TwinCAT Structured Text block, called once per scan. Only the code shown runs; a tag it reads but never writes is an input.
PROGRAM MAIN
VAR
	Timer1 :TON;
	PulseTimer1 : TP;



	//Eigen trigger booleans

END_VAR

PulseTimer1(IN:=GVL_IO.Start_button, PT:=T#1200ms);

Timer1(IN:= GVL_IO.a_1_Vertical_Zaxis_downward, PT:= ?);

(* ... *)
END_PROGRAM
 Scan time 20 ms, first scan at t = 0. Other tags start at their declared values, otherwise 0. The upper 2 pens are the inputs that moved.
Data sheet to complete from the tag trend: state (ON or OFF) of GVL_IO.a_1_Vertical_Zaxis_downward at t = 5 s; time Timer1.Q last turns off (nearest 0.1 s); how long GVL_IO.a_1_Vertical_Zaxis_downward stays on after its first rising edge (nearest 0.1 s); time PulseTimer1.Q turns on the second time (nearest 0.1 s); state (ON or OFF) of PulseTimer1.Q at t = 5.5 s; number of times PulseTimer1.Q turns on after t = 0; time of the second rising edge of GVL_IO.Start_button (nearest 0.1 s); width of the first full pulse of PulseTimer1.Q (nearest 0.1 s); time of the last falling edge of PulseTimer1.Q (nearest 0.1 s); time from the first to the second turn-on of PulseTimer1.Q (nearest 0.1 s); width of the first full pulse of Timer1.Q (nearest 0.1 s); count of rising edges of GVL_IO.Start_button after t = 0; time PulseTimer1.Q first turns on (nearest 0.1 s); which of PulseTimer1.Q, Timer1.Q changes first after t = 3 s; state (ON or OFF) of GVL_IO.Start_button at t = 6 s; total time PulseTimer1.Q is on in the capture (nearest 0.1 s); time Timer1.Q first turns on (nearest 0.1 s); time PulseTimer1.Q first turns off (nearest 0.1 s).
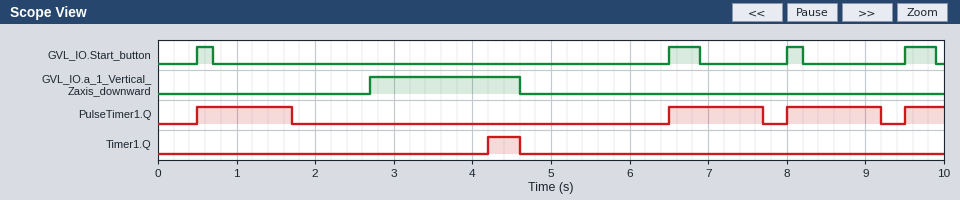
OFF
4.6 s
1.9 s
6.5 s
OFF
4
6.5 s
1.2 s
9.2 s
6.0 s
0.4 s
4
0.5 s
Timer1.Q
OFF
4.1 s
4.2 s
1.7 s
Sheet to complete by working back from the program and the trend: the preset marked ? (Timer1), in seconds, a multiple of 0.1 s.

1.5 s
